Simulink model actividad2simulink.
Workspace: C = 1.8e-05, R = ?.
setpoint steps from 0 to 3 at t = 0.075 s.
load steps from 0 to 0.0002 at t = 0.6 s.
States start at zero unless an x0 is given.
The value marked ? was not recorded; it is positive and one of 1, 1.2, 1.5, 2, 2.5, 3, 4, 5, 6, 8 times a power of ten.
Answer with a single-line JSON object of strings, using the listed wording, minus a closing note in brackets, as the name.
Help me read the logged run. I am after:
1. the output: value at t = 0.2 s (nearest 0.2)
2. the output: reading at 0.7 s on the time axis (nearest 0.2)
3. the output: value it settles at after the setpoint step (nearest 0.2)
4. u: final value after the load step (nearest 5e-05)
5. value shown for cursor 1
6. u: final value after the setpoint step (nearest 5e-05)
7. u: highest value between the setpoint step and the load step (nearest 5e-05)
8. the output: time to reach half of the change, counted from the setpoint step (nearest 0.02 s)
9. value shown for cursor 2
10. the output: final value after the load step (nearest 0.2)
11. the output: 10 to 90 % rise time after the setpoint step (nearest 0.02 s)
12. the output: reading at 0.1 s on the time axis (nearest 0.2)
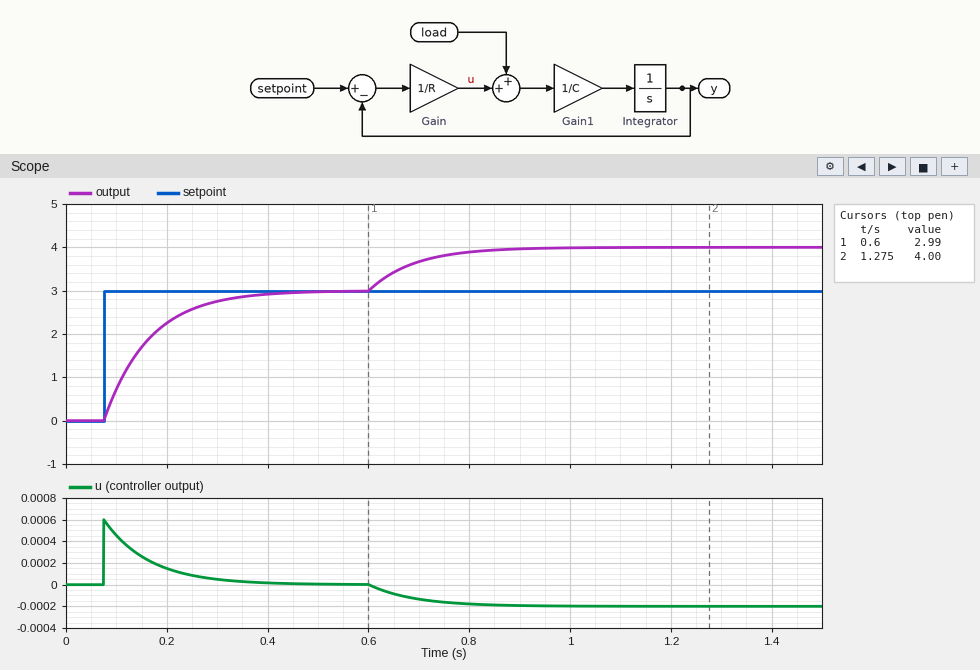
{"the output: value at t = 0.2 s": "2.2", "the output: reading at 0.7 s on the time axis": "3.6", "the output: value it settles at after the setpoint step": "3.0", "u: final value after the load step": "-0.00020", "value shown for cursor 1": "2.99", "u: final value after the setpoint step": "0.00000", "u: highest value between the setpoint step and the load step": "0.00060", "the output: time to reach half of the change, counted from the setpoint step": "0.06 s", "value shown for cursor 2": "4.00", "the output: final value after the load step": "4.0", "the output: 10 to 90 % rise time after the setpoint step": "0.20 s", "the output: reading at 0.1 s on the time axis": "0.8"}
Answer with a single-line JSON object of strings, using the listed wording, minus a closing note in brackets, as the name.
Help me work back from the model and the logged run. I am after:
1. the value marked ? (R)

{"the value marked ?": "5000"}
